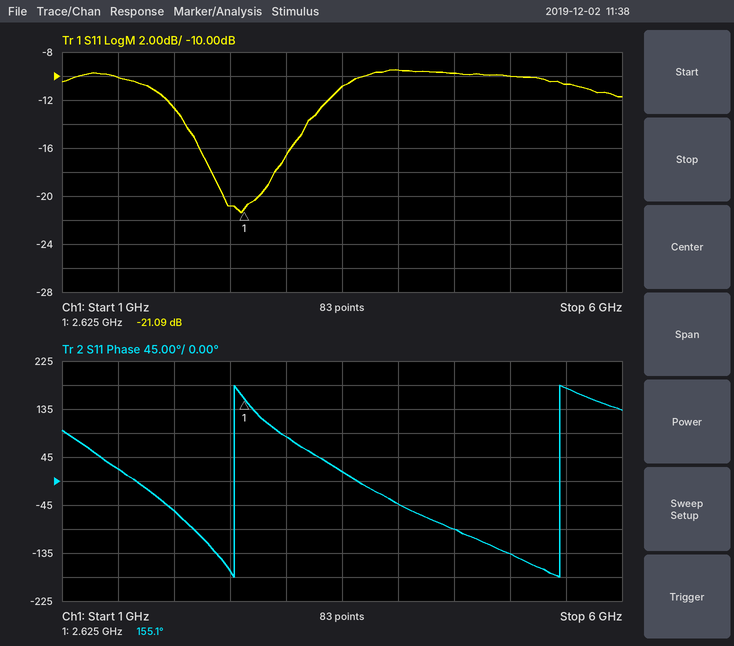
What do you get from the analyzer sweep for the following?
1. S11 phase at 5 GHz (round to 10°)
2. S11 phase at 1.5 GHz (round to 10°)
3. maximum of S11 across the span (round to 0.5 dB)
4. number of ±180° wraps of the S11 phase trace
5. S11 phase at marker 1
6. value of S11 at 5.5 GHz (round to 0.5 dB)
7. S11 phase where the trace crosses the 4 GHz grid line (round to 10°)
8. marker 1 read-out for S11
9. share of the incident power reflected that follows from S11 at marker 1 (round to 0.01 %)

-140°
20°
-9.5 dB
2
155.1°
-10.5 dB
-40°
-21.09 dB
0.78 %
